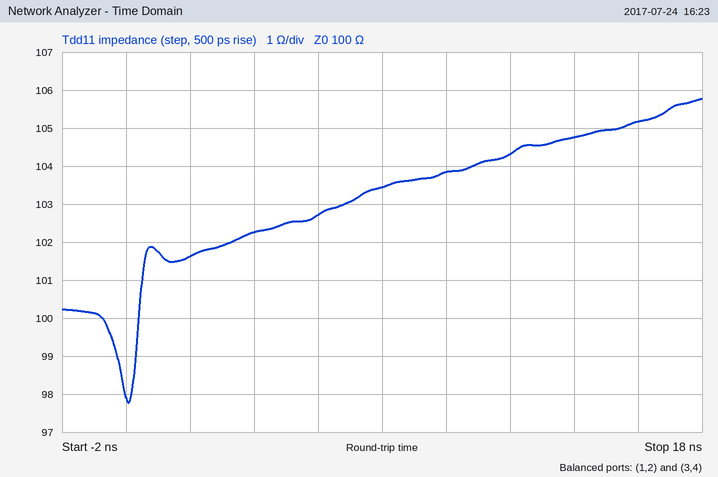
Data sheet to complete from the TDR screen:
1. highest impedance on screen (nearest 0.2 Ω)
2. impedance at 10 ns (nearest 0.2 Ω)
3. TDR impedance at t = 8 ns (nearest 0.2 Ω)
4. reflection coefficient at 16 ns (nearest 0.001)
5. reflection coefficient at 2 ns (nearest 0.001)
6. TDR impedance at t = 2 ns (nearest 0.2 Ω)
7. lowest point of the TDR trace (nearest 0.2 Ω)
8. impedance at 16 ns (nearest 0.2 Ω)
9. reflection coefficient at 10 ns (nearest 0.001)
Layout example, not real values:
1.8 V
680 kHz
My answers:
105.8 Ω
103.8 Ω
103.4 Ω
+0.025
+0.008
101.6 Ω
97.8 Ω
105.2 Ω
+0.019
